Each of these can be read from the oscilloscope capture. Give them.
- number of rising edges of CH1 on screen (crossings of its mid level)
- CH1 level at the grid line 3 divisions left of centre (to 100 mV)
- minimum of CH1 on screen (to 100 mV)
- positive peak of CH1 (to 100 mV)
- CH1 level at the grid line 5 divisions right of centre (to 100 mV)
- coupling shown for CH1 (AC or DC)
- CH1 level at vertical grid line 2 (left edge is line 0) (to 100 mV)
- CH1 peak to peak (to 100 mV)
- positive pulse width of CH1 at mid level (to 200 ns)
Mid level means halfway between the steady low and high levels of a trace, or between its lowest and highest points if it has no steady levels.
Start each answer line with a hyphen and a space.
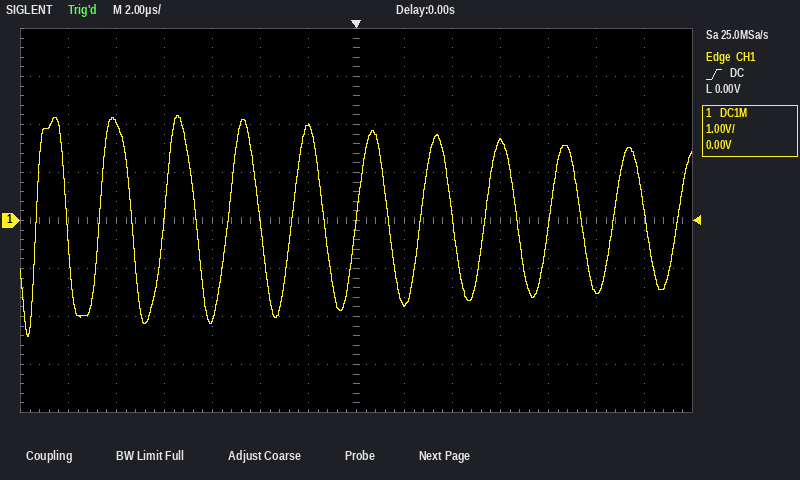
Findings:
- 11
- -2.1 V
- -2.4 V
- 2.2 V
- -1.5 V
- DC
- 2.0 V
- 4.6 V
- 1.4 µs
